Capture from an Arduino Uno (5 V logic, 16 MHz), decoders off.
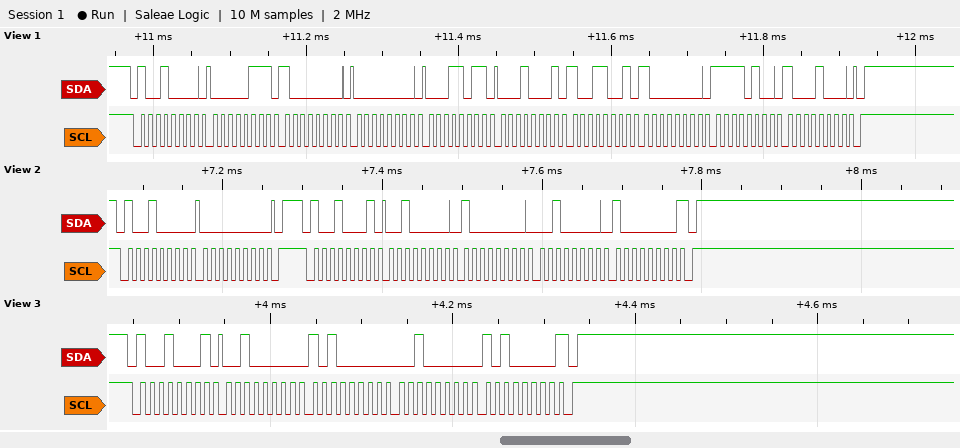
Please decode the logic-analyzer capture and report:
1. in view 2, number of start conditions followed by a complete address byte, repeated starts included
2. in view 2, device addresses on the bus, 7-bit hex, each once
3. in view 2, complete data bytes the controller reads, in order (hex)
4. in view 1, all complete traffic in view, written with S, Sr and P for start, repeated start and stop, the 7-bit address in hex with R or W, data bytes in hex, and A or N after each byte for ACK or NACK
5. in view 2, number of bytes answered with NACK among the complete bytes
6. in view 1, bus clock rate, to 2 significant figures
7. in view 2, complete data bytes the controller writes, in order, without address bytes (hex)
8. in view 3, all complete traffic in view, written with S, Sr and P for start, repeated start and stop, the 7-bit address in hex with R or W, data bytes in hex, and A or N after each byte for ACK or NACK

2
0x48
20 80 20 80
S 48W A 07 A 80 A 00 A 1B A 11 A 99 A 80 A F4 A 88 A P
1
100 kHz
00
S 48R A 20 A A0 A 20 A A0 N P
